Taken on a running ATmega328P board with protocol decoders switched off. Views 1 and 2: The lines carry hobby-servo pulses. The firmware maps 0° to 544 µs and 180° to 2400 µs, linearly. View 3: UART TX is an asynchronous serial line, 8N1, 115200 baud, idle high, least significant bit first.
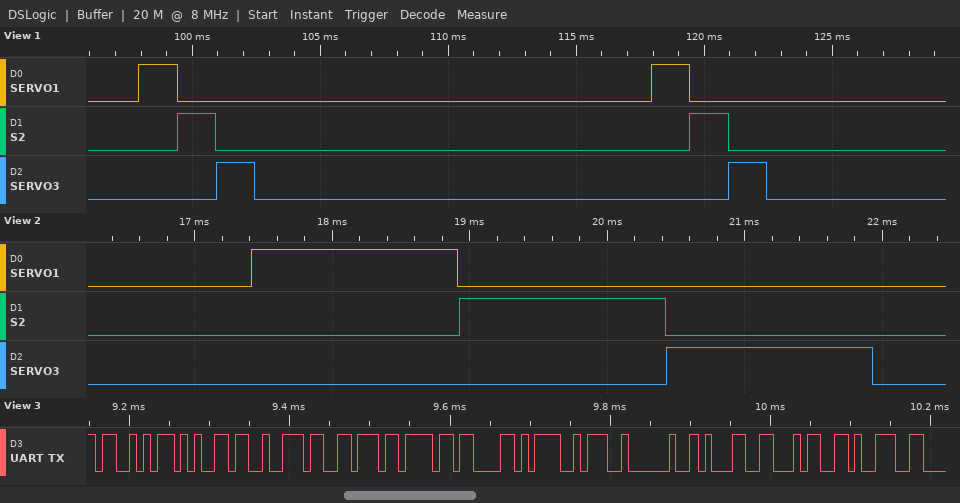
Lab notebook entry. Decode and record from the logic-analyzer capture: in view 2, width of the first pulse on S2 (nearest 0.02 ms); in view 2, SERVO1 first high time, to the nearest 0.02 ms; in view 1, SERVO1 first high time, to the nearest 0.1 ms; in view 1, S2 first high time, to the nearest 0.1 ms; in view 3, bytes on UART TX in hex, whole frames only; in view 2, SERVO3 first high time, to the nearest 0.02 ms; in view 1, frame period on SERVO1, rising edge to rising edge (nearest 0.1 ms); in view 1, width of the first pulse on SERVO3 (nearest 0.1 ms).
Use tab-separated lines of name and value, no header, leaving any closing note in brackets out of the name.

in view 2, width of the first pulse on S2	1.50 ms
in view 2, SERVO1 first high time, to the nearest 0.02 ms	1.50 ms
in view 1, SERVO1 first high time, to the nearest 0.1 ms	1.5 ms
in view 1, S2 first high time, to the nearest 0.1 ms	1.5 ms
in view 3, bytes on UART TX in hex, whole frames only	53 65 72 76 6F 58 3A 20 31 34 39
in view 2, SERVO3 first high time, to the nearest 0.02 ms	1.50 ms
in view 1, frame period on SERVO1, rising edge to rising edge	20.0 ms
in view 1, width of the first pulse on SERVO3	1.5 ms
